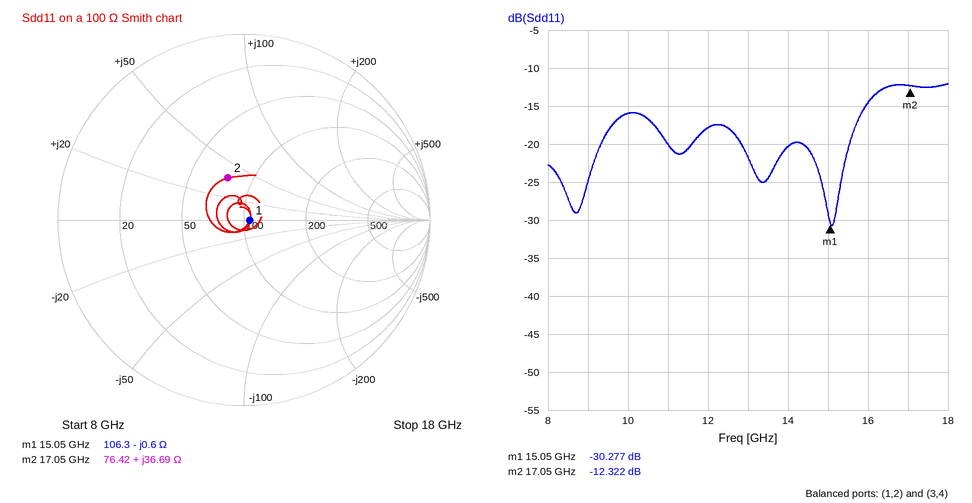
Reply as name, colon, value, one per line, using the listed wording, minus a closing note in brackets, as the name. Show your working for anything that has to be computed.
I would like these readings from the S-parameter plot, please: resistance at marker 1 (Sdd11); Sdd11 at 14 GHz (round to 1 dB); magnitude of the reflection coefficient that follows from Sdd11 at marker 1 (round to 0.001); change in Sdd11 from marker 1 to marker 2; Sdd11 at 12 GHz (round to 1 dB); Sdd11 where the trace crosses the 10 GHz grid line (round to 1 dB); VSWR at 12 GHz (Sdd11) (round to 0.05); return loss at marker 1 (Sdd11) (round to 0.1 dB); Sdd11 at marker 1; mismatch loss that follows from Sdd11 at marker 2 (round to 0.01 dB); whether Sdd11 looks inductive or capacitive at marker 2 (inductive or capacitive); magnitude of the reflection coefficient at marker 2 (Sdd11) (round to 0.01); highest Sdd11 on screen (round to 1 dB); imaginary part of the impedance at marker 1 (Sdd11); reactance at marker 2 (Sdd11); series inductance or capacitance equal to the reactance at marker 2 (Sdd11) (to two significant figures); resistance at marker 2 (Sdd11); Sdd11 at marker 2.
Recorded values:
resistance at marker 1: 106.3 Ω
Sdd11 at 14 GHz: -20 dB
magnitude of the reflection coefficient that follows from Sdd11 at marker 1: 10^(-30.277/20) ≈ 0.031
change in Sdd11 from marker 1 to marker 2: -12.322 − (-30.277) = 17.955 dB
Sdd11 at 12 GHz: -18 dB
Sdd11 where the trace crosses the 10 GHz grid line: -16 dB
VSWR at 12 GHz (Sdd11): |Γ| = 10^(-18/20) = 0.1259; VSWR = (1 + 0.1259)/(1 − 0.1259) ≈ 1.29, so 1.30 to the nearest 0.05
return loss at marker 1 (Sdd11): 30.3 dB
Sdd11 at marker 1: -30.277 dB
mismatch loss that follows from Sdd11 at marker 2: −10 log10(1 − 10^(-12.322/10)) ≈ 0.26 dB
whether Sdd11 looks inductive or capacitive at marker 2: inductive
magnitude of the reflection coefficient at marker 2 (Sdd11): 0.24
highest Sdd11 on screen: -12 dB
imaginary part of the impedance at marker 1: -0.6 Ω
reactance at marker 2: +36.69 Ω
series inductance or capacitance equal to the reactance at marker 2 (Sdd11): L = 36.69 Ω/(2π × 17.05 GHz) ≈ 342 pH, so 340 pH to two significant figures
resistance at marker 2: 76.42 Ω
Sdd11 at marker 2: -12.322 dB
